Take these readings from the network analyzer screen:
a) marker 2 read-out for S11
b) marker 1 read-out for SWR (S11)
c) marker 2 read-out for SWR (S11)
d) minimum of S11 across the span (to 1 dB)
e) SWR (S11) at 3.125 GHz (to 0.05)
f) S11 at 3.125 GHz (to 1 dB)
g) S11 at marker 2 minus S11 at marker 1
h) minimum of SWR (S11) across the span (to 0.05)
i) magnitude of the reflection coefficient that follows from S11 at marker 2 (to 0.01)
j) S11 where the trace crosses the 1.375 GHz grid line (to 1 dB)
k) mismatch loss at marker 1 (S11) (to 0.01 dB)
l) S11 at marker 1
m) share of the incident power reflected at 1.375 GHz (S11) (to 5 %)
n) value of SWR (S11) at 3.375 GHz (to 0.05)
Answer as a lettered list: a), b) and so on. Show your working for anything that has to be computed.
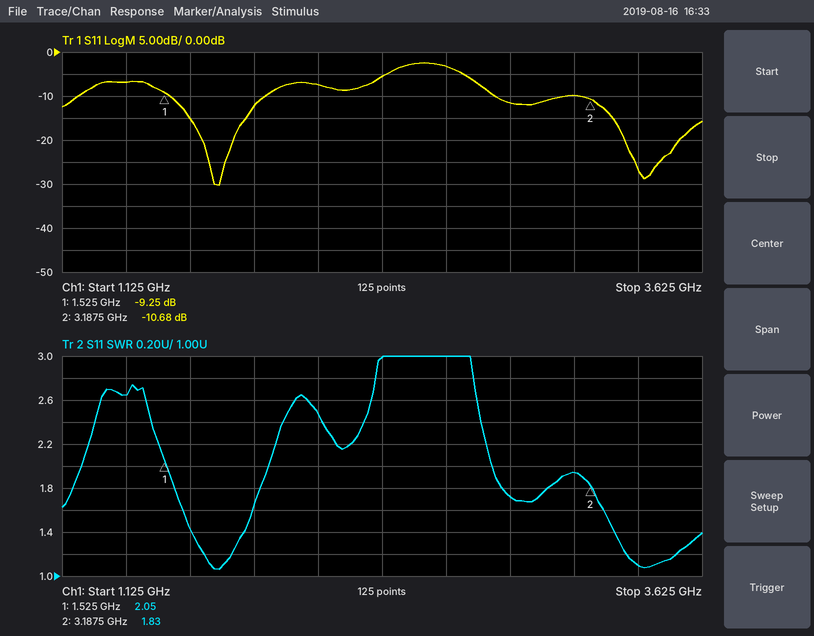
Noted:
a) -10.68 dB
b) 2.05
c) 1.83
d) -30 dB
e) 1.95
f) -10 dB
g) -10.68 − (-9.25) = -1.43 dB
h) 1.05
i) 10^(-10.68/20) ≈ 0.29
j) -7 dB
k) −10 log10(1 − 10^(-9.25/10)) ≈ 0.55 dB
l) -9.25 dB
m) 10^(-7/10) ≈ 20 %
n) 1.10
